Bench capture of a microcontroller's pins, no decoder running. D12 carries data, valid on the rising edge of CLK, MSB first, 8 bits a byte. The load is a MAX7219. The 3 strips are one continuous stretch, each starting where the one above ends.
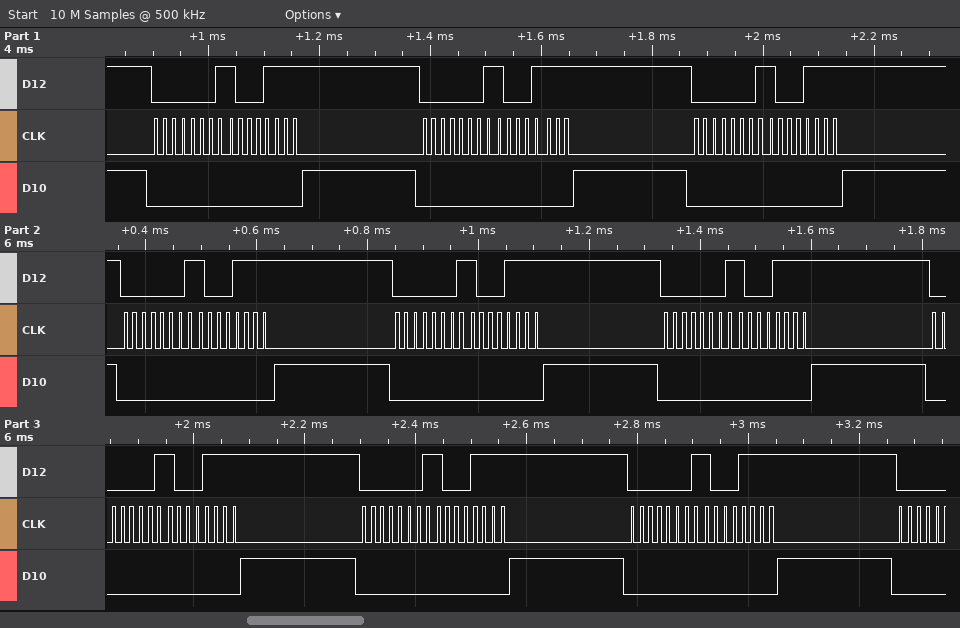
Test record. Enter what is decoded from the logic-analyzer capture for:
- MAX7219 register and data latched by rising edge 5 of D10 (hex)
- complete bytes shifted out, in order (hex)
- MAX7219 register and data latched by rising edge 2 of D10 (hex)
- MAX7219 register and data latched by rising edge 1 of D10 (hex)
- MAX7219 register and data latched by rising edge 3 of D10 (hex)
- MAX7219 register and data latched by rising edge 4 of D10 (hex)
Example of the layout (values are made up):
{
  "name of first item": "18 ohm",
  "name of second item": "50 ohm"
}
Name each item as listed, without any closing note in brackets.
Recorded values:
{
  "MAX7219 register and data latched by rising edge 5 of D10": "register 0x1, data 0x8F",
  "complete bytes shifted out, in order": "01 8F 01 8F 01 8F 01 8F 01 8F 01 8F 01 8F 01 8F 01 8F",
  "MAX7219 register and data latched by rising edge 2 of D10": "register 0x1, data 0x8F",
  "MAX7219 register and data latched by rising edge 1 of D10": "register 0x1, data 0x8F",
  "MAX7219 register and data latched by rising edge 3 of D10": "register 0x1, data 0x8F",
  "MAX7219 register and data latched by rising edge 4 of D10": "register 0x1, data 0x8F"
}
